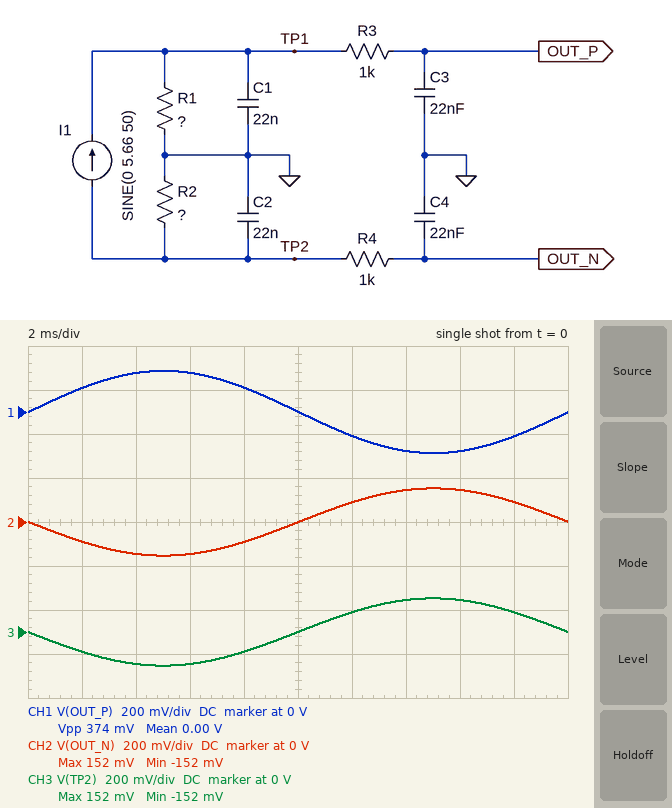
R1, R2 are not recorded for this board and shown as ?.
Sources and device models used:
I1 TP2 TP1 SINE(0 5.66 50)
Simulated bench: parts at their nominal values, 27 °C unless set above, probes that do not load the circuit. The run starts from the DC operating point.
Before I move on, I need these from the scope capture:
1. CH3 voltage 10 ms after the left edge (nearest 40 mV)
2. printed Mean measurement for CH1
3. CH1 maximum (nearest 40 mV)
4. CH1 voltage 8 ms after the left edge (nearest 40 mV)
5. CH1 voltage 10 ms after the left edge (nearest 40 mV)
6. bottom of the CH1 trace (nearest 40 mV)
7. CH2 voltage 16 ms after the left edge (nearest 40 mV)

0 V
0.00 V
200 mV
120 mV
0 V
-200 mV
160 mV
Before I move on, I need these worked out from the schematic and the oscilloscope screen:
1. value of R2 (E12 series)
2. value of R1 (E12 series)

0.027 Ω
0.033 Ω
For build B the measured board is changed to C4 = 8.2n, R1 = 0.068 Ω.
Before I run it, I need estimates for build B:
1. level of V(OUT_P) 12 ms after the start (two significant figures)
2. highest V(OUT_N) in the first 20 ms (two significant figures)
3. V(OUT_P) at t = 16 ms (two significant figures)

-220 mV
150 mV
-370 mV
